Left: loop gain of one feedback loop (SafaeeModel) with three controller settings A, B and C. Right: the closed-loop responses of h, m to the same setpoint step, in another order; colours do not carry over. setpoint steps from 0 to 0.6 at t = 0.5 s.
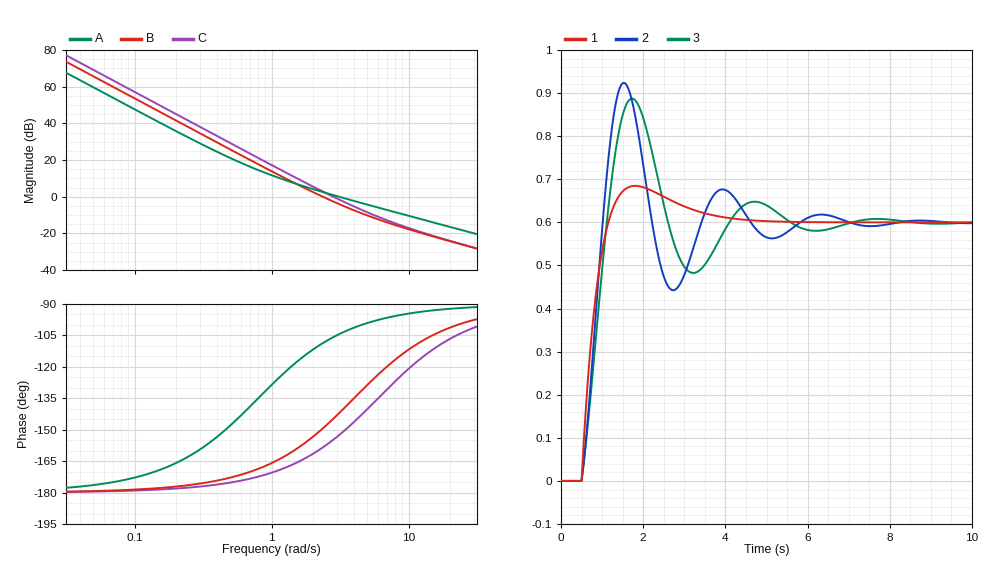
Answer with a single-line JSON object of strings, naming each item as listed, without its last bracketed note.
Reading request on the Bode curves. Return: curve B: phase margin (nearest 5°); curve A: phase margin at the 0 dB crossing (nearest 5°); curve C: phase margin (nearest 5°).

{"curve B: phase margin": "30°", "curve A: phase margin at the 0 dB crossing": "75°", "curve C: phase margin": "25°"}
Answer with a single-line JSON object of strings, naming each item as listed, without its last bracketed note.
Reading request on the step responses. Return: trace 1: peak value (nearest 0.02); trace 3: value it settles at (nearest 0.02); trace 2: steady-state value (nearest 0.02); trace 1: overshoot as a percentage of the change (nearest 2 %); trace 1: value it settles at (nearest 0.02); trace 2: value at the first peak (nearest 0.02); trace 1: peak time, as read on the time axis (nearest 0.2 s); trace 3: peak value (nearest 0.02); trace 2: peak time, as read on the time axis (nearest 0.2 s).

{"trace 1: peak value": "0.68", "trace 3: value it settles at": "0.60", "trace 2: steady-state value": "0.60", "trace 1: overshoot as a percentage of the change": "14 %", "trace 1: value it settles at": "0.60", "trace 2: value at the first peak": "0.92", "trace 1: peak time, as read on the time axis": "1.8 s", "trace 3: peak value": "0.88", "trace 2: peak time, as read on the time axis": "1.6 s"}
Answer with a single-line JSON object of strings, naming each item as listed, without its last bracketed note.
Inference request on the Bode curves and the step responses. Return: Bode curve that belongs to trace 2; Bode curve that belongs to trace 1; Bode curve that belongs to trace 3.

{"Bode curve that belongs to trace 2": "C", "Bode curve that belongs to trace 1": "A", "Bode curve that belongs to trace 3": "B"}
